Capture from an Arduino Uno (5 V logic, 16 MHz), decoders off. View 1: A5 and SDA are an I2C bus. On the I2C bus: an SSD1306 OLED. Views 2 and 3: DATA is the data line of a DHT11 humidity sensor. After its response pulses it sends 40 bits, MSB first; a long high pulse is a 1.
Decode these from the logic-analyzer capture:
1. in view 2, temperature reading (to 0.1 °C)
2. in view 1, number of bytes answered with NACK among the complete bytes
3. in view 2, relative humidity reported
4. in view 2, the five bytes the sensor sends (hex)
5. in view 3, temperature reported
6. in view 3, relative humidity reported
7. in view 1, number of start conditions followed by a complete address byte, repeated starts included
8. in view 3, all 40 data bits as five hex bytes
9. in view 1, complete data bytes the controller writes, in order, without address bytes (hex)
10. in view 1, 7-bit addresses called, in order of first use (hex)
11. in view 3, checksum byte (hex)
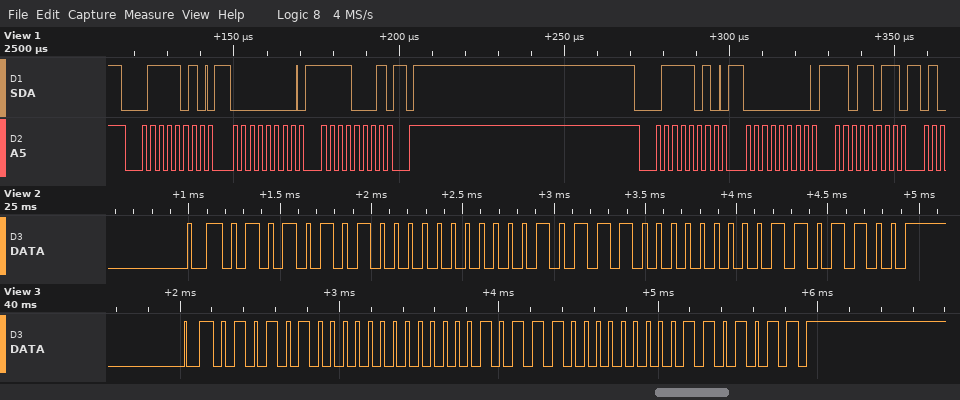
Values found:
23.0 °C
0
85 %
55 00 17 00 6C
23.0 °C
84 %
2
54 00 17 00 6B
00 F1 00 DB
0x3D
0x6B
